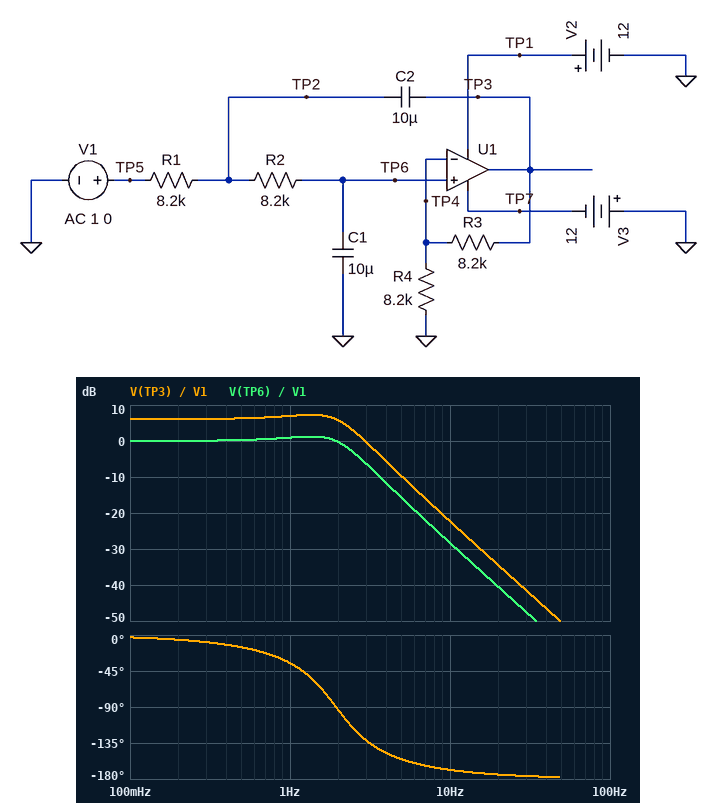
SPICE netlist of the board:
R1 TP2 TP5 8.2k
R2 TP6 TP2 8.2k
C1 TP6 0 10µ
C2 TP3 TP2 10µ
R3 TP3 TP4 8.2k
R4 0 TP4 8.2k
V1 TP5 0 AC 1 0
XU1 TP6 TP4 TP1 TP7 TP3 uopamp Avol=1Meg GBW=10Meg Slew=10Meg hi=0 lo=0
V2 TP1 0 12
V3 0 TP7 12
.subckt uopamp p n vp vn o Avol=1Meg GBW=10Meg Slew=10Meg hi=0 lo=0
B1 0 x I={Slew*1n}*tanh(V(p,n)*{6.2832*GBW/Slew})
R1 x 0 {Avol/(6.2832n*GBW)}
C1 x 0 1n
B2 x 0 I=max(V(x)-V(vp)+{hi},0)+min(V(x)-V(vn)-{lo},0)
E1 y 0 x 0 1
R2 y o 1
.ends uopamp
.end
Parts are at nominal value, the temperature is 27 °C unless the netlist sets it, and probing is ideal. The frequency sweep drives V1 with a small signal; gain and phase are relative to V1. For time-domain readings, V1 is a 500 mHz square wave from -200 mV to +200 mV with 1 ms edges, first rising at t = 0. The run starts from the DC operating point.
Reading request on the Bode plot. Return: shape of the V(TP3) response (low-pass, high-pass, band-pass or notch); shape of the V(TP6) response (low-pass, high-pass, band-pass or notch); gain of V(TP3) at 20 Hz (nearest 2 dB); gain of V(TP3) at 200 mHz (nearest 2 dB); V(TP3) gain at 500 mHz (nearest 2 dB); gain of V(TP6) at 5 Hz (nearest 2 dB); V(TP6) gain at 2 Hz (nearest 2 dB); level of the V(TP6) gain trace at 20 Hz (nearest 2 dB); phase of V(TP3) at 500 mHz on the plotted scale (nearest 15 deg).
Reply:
low-pass
low-pass
-34 dB
6 dB
6 dB
-16 dB
0 dB
-40 dB
-15 deg
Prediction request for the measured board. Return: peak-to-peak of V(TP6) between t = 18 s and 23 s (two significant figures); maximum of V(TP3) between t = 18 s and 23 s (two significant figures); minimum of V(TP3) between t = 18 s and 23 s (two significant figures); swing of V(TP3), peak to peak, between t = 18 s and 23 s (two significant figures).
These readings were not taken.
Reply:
530 mV
530 mV
-530 mV
1.1 V
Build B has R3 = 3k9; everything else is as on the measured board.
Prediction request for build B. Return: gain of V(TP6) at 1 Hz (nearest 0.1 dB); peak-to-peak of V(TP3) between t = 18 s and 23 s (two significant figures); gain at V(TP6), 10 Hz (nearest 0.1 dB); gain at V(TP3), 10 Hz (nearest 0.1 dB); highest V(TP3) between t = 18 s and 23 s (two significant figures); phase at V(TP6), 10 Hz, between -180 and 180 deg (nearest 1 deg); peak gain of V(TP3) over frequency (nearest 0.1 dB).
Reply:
-0.6 dB
620 mV
-28.5 dB
-25.2 dB
310 mV
-163 deg
3.4 dB
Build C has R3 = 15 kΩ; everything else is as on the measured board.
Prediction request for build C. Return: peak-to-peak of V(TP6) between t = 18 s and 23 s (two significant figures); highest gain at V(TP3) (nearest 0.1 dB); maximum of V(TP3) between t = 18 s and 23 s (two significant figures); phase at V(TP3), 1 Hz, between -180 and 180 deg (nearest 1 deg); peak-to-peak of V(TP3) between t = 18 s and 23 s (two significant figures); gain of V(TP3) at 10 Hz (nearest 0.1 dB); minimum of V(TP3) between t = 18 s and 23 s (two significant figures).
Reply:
860 mV
24.4 dB
1.2 V
-7 deg
2.4 V
-19.1 dB
-1.2 V
